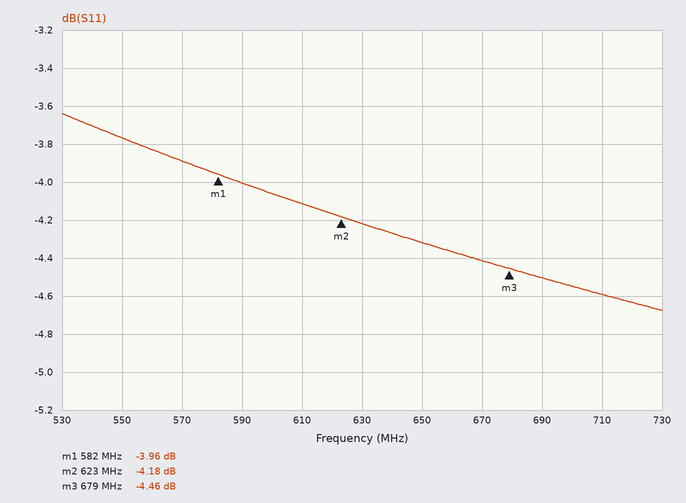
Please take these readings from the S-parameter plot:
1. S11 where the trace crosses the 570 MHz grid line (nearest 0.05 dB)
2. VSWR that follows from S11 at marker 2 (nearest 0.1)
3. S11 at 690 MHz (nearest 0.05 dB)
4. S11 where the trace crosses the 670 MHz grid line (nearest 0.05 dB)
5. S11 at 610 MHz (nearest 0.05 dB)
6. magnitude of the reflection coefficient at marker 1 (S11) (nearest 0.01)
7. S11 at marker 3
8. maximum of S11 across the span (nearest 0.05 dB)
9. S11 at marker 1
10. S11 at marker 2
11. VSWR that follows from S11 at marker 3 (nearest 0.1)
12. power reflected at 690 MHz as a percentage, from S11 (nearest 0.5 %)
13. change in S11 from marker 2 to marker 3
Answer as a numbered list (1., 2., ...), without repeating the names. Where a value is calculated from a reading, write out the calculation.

1. -3.90 dB
2. (1 + 0.6180)/(1 − 0.6180) ≈ 4.2
3. -4.50 dB
4. -4.40 dB
5. -4.10 dB
6. 10^(-3.96/20) ≈ 0.63
7. -4.46 dB
8. -3.65 dB
9. -3.96 dB
10. -4.18 dB
11. (1 + 0.5984)/(1 − 0.5984) ≈ 4.0
12. 10^(-4.5/10) ≈ 35.5 %
13. -4.46 − (-4.18) = -0.28 dB
